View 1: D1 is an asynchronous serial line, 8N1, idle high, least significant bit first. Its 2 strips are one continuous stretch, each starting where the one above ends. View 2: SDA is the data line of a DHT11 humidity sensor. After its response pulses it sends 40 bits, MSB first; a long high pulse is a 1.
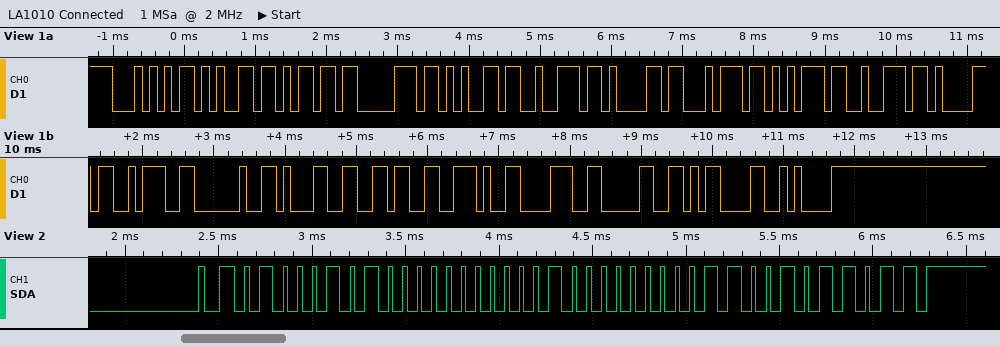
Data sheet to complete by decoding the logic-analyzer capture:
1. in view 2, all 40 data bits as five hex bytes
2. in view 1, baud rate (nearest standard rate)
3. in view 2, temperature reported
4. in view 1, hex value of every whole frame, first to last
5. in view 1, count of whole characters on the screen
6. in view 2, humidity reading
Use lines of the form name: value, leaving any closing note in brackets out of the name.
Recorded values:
in view 2, all 40 data bits as five hex bytes: 45 00 10 06 5B
in view 1, baud rate: 9600 baud
in view 2, temperature reported: 16.6 °C
in view 1, hex value of every whole frame, first to last: 0x54 0x65 0x6D 0x70 0x65 0x72 0x61 0x74 0x75 0x72 0x61 0x3A 0x20 0x31 0x36 0x2E 0x38 0x30 0x0D 0x0A
in view 1, count of whole characters on the screen: 20
in view 2, humidity reading: 69 %
